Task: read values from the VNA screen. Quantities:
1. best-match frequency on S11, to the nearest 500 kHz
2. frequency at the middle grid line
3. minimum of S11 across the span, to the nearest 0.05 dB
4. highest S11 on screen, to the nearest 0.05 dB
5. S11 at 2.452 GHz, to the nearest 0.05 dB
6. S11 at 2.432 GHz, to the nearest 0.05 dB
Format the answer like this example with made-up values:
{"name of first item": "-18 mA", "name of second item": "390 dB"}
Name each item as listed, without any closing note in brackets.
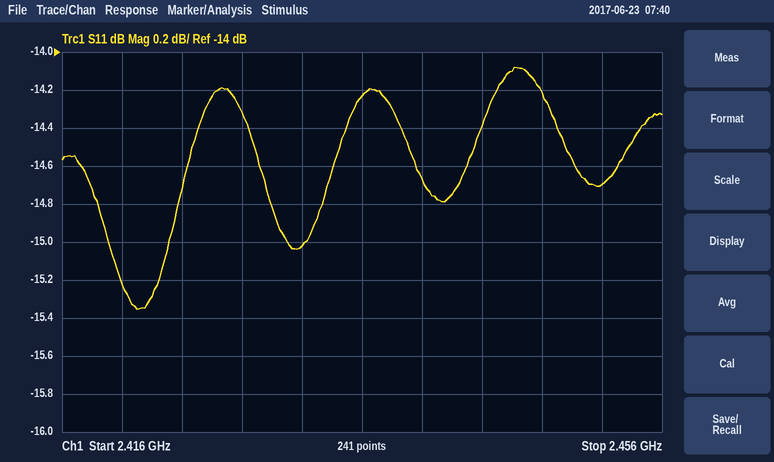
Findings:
{"best-match frequency on S11, to the nearest 500 kHz": "2.4210 GHz", "frequency at the middle grid line": "2.436 GHz", "minimum of S11 across the span, to the nearest 0.05 dB": "-15.35 dB", "highest S11 on screen, to the nearest 0.05 dB": "-14.10 dB", "S11 at 2.452 GHz, to the nearest 0.05 dB": "-14.70 dB", "S11 at 2.432 GHz, to the nearest 0.05 dB": "-15.00 dB"}
